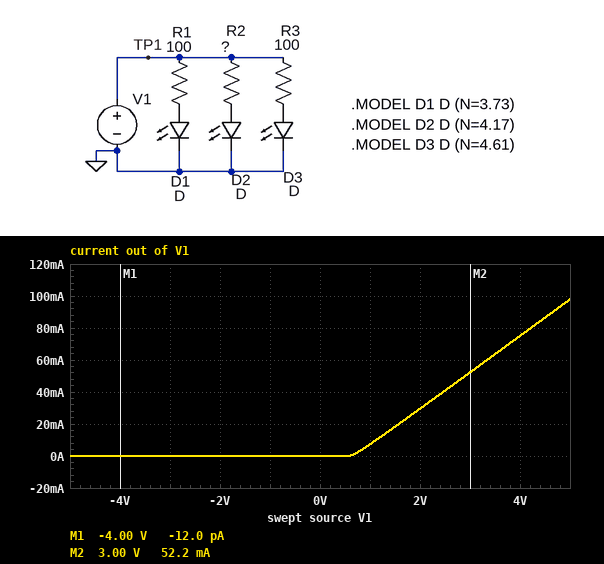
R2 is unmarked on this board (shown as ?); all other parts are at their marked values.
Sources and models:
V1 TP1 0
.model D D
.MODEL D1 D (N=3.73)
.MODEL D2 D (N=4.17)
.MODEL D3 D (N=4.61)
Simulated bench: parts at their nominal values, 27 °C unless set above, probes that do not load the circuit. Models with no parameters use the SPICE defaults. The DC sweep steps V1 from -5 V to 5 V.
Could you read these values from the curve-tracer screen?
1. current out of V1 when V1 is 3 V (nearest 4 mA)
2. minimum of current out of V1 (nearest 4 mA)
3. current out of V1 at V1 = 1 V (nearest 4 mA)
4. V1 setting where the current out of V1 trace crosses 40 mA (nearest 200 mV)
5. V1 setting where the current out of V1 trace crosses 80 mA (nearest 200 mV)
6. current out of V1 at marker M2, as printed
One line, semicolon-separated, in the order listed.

52 mA; 0 A; 8 mA; 2.4 V; 4.2 V; 52.2 mA
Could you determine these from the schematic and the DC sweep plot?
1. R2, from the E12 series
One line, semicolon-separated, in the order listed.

330 Ω
